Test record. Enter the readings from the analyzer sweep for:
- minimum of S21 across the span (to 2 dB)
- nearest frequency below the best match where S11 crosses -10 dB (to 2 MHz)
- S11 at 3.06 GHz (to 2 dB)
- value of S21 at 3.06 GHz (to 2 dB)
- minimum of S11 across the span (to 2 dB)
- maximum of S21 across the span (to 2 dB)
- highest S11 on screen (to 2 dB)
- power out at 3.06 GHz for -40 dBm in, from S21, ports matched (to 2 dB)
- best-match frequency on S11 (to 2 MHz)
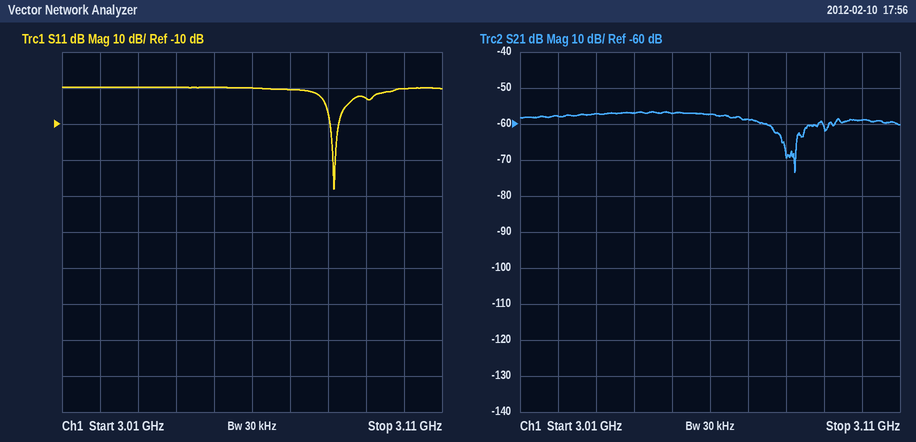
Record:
-74 dB
3.080 GHz
0 dB
-58 dB
-28 dB
-56 dB
0 dB
-98 dBm
3.082 GHz
